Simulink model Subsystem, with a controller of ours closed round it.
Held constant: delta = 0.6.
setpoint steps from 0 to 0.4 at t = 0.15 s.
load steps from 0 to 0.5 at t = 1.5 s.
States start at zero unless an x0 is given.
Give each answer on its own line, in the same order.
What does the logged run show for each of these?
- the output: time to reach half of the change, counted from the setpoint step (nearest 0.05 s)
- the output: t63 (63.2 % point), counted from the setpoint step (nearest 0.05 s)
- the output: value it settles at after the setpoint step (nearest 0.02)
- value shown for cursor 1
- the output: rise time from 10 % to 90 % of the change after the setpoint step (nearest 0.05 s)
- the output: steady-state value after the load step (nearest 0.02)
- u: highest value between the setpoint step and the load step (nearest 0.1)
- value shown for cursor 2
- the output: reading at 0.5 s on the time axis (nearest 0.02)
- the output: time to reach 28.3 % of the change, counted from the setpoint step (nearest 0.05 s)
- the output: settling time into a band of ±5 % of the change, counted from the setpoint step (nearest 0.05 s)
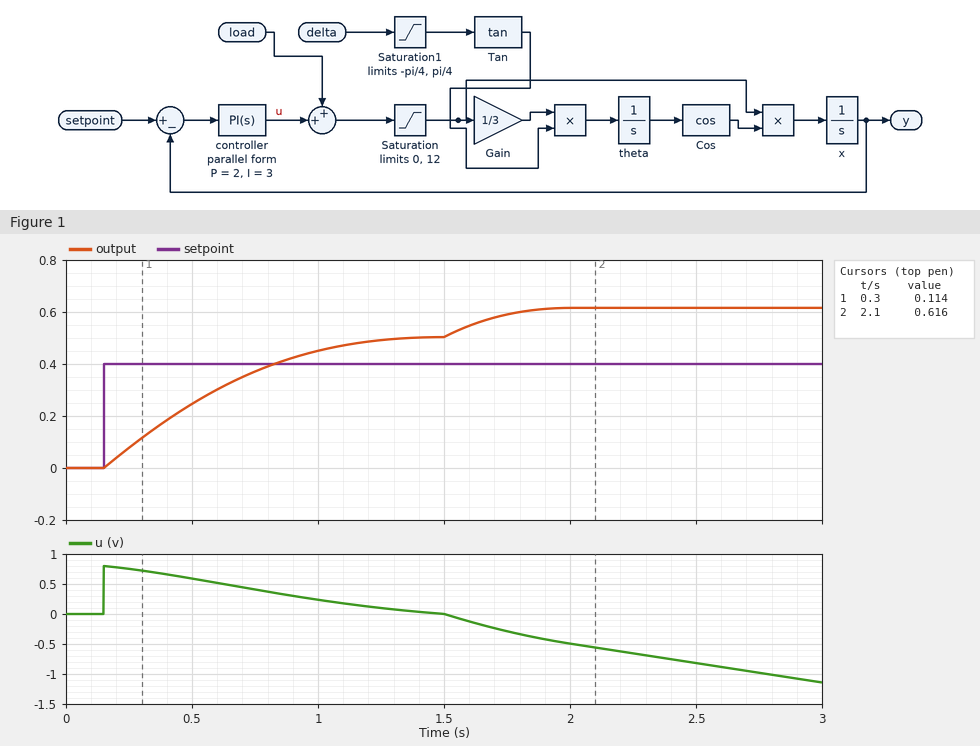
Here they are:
0.35 s
0.50 s
0.50
0.114
0.80 s
0.62
0.8
0.616
0.24
0.20 s
1.00 s
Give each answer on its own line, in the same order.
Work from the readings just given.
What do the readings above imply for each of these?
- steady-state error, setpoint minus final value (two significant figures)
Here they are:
-0.10
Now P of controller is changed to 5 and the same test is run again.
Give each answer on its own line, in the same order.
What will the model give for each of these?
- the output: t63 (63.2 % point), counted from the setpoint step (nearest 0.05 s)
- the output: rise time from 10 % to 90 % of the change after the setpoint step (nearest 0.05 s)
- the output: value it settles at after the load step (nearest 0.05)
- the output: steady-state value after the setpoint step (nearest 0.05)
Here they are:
0.20 s
0.45 s
0.50
0.45
